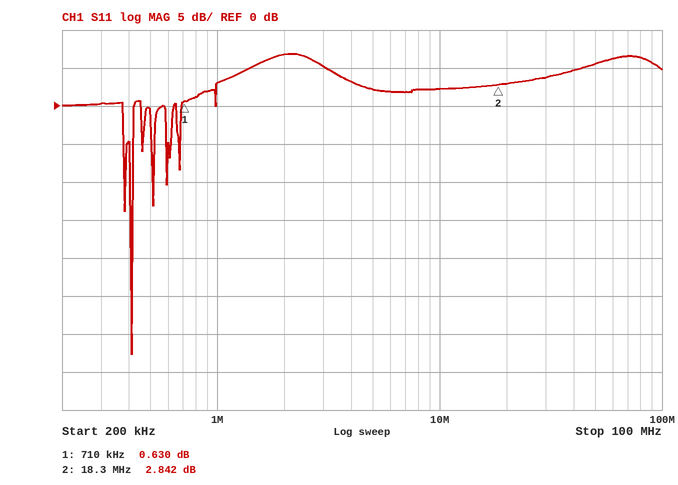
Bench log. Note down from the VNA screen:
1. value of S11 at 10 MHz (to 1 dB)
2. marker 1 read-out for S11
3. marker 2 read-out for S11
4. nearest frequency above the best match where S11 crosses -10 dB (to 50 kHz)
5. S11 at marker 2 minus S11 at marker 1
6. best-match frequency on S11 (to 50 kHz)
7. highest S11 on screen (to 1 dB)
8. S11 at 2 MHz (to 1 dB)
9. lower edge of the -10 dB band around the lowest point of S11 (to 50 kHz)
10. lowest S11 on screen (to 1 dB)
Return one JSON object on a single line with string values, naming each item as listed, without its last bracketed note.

{"value of S11 at 10 MHz": "2 dB", "marker 1 read-out for S11": "0.630 dB", "marker 2 read-out for S11": "2.842 dB", "nearest frequency above the best match where S11 crosses -10 dB": "400 kHz", "S11 at marker 2 minus S11 at marker 1": "2.212 dB", "best-match frequency on S11": "400 kHz", "highest S11 on screen": "7 dB", "S11 at 2 MHz": "7 dB", "lower edge of the -10 dB band around the lowest point of S11": "400 kHz", "lowest S11 on screen": "-33 dB"}
